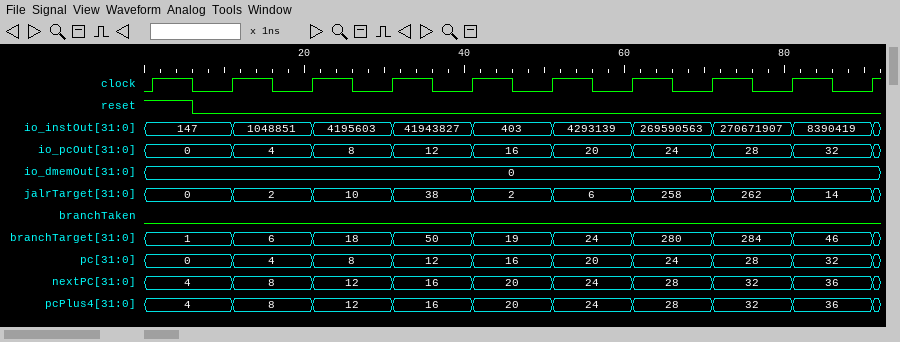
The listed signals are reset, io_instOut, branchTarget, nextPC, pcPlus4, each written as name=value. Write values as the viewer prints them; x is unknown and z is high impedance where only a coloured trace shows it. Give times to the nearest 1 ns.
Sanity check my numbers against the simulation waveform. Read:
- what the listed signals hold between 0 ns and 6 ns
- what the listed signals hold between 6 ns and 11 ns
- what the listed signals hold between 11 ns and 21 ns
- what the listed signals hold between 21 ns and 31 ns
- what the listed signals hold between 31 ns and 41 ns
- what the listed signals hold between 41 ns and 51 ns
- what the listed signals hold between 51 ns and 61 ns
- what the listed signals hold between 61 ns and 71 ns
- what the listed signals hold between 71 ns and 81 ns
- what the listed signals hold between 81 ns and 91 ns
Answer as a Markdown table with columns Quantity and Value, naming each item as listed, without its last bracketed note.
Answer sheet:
| Quantity | Value |
|---|---|
| what the listed signals hold between 0 ns and 6 ns | reset=1, io_instOut=147, branchTarget=1, nextPC=4, pcPlus4=4 |
| what the listed signals hold between 6 ns and 11 ns | reset=0, io_instOut=147, branchTarget=1, nextPC=4, pcPlus4=4 |
| what the listed signals hold between 11 ns and 21 ns | reset=0, io_instOut=1048851, branchTarget=6, nextPC=8, pcPlus4=8 |
| what the listed signals hold between 21 ns and 31 ns | reset=0, io_instOut=4195603, branchTarget=18, nextPC=12, pcPlus4=12 |
| what the listed signals hold between 31 ns and 41 ns | reset=0, io_instOut=41943827, branchTarget=50, nextPC=16, pcPlus4=16 |
| what the listed signals hold between 41 ns and 51 ns | reset=0, io_instOut=403, branchTarget=19, nextPC=20, pcPlus4=20 |
| what the listed signals hold between 51 ns and 61 ns | reset=0, io_instOut=4293139, branchTarget=24, nextPC=24, pcPlus4=24 |
| what the listed signals hold between 61 ns and 71 ns | reset=0, io_instOut=269590563, branchTarget=280, nextPC=28, pcPlus4=28 |
| what the listed signals hold between 71 ns and 81 ns | reset=0, io_instOut=270671907, branchTarget=284, nextPC=32, pcPlus4=32 |
| what the listed signals hold between 81 ns and 91 ns | reset=0, io_instOut=8390419, branchTarget=46, nextPC=36, pcPlus4=36 |
